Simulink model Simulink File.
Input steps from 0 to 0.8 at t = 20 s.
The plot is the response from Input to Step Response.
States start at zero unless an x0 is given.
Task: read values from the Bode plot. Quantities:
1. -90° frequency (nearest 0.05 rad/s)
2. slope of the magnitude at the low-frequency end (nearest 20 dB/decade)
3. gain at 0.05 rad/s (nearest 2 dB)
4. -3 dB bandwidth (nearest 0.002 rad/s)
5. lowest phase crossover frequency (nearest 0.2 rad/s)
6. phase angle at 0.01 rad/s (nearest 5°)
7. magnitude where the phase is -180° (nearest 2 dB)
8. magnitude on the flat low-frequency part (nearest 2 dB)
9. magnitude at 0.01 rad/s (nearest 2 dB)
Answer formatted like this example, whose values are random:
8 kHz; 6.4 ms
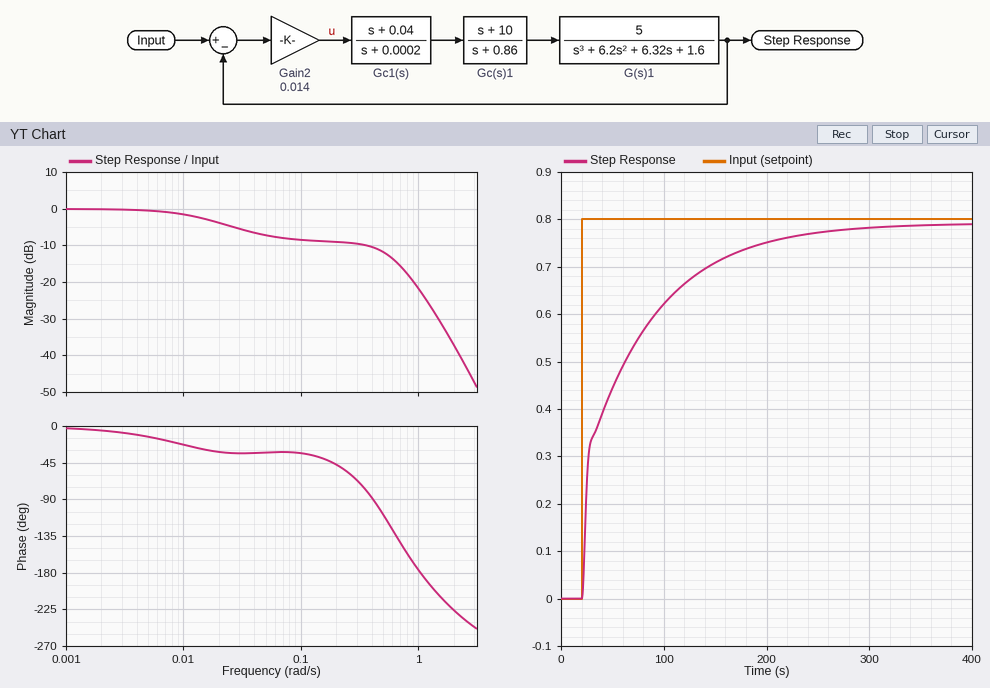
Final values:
0.40 rad/s; 0 dB/decade; -8 dB; 0.016 rad/s; 1.0 rad/s; -25°; -22 dB; 0 dB; -2 dB
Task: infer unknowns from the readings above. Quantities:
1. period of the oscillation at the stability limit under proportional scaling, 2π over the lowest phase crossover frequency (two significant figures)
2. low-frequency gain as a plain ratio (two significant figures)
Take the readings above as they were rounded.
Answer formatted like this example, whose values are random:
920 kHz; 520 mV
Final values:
6.3 s; 1.0
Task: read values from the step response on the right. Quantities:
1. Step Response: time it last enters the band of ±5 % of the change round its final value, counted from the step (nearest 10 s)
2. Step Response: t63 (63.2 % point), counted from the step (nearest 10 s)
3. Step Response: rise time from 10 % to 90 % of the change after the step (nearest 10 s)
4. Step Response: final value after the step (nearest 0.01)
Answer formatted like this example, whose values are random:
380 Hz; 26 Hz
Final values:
180 s; 40 s; 130 s; 0.79
